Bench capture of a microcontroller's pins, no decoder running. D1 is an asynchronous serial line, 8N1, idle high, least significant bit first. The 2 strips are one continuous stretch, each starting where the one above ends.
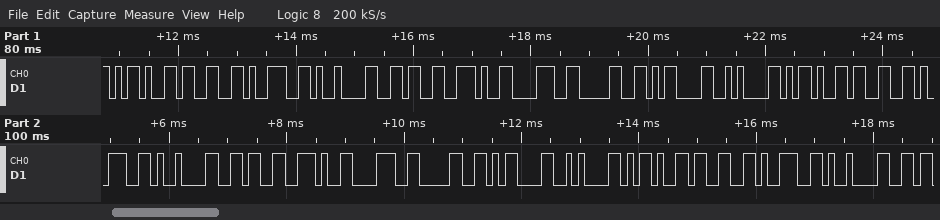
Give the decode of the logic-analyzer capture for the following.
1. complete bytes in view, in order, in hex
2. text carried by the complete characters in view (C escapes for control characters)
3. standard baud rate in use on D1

2D 33 39 09 36 2E 38 30 0D 0A 2D 33 39 09 36 2E 38 30 0D 0A 2D 33 39 09
"-39\t6.80\r\n-39\t6.80\r\n-39\t"
9600 baud
